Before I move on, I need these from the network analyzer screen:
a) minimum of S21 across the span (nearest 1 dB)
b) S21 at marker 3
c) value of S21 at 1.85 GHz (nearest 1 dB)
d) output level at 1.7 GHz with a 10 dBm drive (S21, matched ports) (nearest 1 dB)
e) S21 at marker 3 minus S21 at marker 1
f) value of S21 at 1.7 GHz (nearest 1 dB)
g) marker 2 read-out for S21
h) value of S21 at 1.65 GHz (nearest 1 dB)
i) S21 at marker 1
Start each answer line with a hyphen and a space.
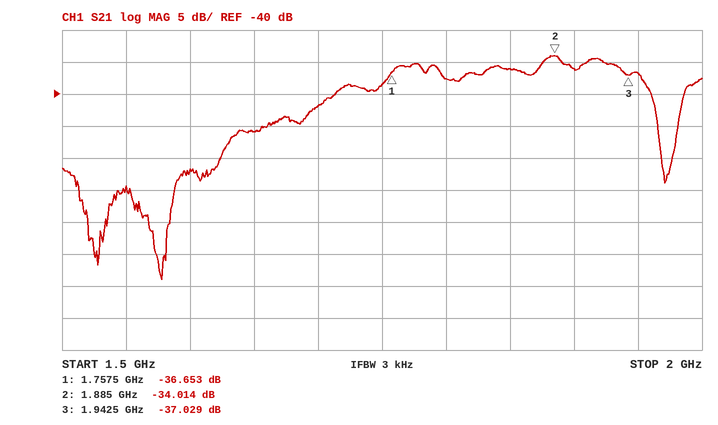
- -69 dB
- -37.029 dB
- -36 dB
- -32 dBm
- -0.376 dB
- -42 dB
- -34.014 dB
- -46 dB
- -36.653 dB
